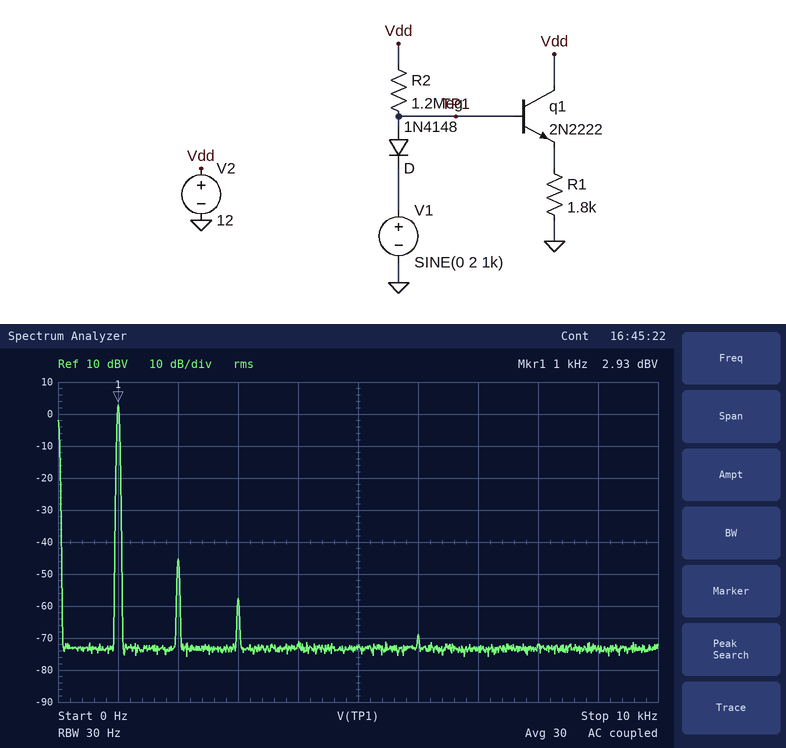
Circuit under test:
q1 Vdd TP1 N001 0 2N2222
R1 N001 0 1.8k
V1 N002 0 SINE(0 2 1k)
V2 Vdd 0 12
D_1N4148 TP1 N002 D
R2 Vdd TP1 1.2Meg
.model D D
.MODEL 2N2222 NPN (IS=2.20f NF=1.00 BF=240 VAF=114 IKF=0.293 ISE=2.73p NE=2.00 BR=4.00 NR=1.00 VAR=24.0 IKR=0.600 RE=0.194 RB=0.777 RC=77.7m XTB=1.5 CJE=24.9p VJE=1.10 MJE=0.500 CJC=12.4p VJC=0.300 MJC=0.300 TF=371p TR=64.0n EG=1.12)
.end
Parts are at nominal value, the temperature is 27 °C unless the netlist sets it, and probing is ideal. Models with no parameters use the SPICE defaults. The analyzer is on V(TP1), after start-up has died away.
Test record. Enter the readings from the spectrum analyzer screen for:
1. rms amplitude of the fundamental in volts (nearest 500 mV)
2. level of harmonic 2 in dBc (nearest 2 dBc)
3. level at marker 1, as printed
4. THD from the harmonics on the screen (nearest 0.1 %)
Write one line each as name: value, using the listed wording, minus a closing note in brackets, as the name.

rms amplitude of the fundamental in volts: 1.5 V
level of harmonic 2 in dBc: -48 dBc
level at marker 1, as printed: 2.93 dBV
THD from the harmonics on the screen: 0.4 %
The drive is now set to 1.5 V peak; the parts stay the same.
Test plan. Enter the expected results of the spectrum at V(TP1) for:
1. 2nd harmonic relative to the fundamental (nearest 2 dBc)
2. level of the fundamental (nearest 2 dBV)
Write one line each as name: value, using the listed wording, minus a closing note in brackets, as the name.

2nd harmonic relative to the fundamental: -50 dBc
level of the fundamental: 0 dBV
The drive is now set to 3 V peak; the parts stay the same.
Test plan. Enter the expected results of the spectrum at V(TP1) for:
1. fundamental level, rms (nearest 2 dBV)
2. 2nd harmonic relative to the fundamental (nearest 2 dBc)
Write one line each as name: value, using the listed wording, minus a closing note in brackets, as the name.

fundamental level, rms: 6 dBV
2nd harmonic relative to the fundamental: -30 dBc
